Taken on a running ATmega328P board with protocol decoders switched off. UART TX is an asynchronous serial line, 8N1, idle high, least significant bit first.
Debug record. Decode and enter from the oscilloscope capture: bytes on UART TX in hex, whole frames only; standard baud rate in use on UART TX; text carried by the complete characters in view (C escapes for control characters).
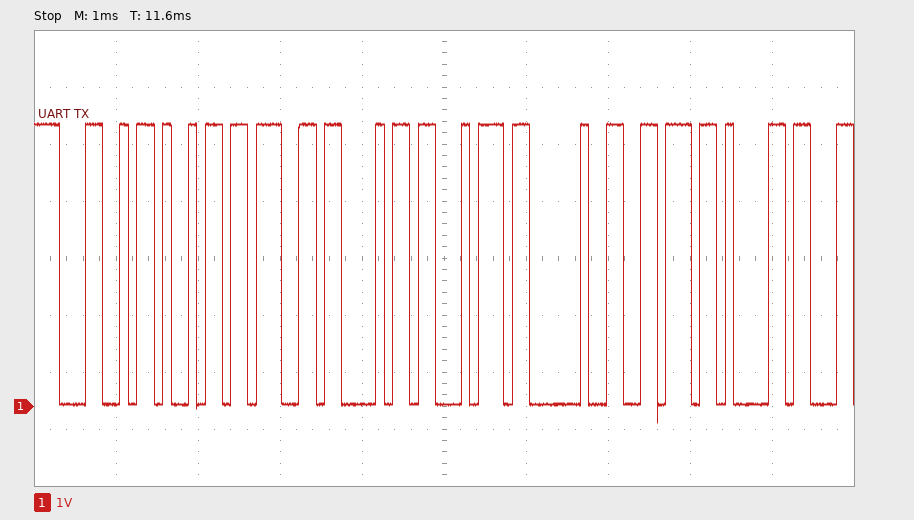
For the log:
0x4C 0x69 0x67 0x68 0x74 0x20 0x76 0x61
9600 baud
"Light va"
